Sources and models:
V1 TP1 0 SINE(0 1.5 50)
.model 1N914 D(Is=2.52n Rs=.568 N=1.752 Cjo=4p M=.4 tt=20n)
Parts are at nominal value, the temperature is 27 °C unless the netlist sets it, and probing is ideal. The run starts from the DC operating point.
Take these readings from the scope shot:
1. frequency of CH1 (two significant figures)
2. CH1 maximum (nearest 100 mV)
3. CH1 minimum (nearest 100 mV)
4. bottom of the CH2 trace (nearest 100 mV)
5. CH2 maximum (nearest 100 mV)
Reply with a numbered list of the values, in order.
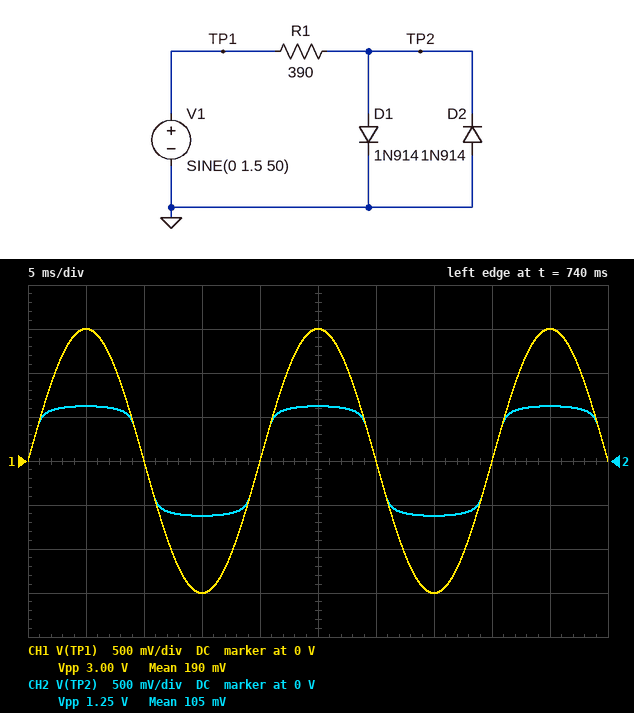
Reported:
1. 50 Hz
2. 1.5 V
3. -1.5 V
4. -600 mV
5. 600 mV
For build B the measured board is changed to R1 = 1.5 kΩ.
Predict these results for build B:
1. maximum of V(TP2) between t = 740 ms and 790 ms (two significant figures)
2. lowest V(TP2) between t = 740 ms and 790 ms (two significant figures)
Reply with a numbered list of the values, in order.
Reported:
1. 560 mV
2. -560 mV
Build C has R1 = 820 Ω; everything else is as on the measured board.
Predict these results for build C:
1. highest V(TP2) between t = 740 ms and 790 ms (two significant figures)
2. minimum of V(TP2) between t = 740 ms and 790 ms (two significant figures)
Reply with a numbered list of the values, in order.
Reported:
1. 590 mV
2. -590 mV
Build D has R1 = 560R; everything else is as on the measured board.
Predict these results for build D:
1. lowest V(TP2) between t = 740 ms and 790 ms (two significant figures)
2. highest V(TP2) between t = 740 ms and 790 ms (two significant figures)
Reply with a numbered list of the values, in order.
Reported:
1. -610 mV
2. 610 mV
